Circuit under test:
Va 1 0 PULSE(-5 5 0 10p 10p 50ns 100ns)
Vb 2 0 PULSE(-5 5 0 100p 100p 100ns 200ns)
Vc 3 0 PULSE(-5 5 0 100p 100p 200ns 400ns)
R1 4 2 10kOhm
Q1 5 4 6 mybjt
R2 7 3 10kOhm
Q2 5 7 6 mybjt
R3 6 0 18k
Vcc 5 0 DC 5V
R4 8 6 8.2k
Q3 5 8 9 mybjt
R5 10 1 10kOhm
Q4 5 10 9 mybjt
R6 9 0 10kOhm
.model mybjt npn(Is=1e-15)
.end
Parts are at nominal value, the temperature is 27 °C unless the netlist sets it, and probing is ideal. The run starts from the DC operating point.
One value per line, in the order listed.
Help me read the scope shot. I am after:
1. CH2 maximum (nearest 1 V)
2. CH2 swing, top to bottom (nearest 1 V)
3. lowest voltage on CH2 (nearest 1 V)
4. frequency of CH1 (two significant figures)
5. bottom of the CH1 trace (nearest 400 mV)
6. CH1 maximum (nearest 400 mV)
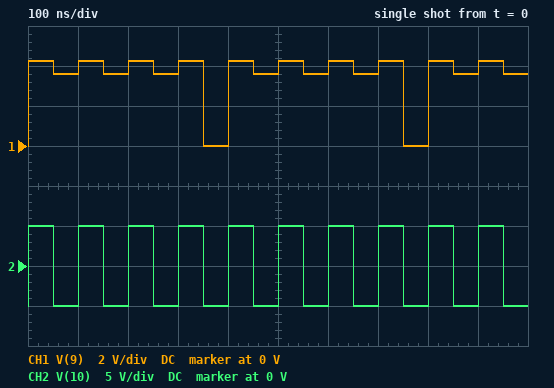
5 V
10 V
-5 V
2.5 MHz
0 V
4.4 V
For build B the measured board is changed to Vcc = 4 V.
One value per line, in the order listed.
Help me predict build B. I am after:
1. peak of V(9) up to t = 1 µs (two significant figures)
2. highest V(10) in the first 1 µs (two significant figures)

3.9 V
4.6 V
